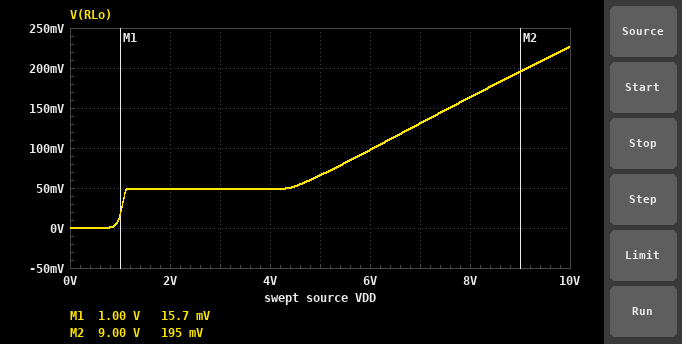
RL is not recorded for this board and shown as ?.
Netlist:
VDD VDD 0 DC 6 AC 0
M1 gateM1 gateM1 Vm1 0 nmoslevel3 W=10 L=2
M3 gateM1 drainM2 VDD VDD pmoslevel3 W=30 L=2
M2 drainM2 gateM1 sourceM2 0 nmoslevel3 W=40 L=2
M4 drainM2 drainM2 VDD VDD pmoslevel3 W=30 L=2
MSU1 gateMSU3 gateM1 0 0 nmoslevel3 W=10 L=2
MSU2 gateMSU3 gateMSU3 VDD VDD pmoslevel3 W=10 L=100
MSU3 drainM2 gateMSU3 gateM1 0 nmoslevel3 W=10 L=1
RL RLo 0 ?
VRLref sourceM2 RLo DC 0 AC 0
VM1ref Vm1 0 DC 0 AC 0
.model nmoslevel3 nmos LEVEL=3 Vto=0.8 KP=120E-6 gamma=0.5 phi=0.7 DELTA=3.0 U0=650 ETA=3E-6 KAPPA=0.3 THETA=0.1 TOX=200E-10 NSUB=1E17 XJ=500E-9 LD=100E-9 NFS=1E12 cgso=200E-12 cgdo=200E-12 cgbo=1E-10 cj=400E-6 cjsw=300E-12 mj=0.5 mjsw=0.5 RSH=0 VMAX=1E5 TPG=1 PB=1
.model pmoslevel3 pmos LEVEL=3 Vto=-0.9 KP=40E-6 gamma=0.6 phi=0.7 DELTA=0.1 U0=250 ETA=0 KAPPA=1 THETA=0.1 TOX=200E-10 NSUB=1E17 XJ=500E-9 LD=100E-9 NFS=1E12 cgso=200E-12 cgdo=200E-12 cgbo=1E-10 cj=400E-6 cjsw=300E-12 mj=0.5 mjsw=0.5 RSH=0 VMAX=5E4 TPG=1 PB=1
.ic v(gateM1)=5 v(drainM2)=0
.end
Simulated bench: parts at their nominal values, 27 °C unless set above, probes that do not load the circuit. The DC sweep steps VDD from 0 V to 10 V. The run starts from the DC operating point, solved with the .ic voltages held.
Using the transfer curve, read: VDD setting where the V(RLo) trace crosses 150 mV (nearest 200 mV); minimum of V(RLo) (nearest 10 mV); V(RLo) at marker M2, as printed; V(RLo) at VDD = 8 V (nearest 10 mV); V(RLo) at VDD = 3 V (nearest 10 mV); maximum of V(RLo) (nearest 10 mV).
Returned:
7.6 V
0 V
195 mV
160 mV
50 mV
230 mV
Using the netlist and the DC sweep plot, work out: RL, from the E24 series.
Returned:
12 kΩ
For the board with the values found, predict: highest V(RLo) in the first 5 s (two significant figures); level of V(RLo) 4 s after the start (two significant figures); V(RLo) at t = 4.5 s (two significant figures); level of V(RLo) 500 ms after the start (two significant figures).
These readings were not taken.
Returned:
44 mV
33 mV
39 mV
3.0 mV
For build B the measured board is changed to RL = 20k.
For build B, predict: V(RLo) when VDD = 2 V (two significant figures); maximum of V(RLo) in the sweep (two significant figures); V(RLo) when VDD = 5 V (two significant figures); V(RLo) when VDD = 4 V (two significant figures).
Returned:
46 mV
250 mV
73 mV
48 mV
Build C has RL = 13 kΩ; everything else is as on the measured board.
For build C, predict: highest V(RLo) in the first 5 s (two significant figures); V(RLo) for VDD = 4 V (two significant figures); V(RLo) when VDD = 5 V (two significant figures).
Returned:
44 mV
45 mV
67 mV
